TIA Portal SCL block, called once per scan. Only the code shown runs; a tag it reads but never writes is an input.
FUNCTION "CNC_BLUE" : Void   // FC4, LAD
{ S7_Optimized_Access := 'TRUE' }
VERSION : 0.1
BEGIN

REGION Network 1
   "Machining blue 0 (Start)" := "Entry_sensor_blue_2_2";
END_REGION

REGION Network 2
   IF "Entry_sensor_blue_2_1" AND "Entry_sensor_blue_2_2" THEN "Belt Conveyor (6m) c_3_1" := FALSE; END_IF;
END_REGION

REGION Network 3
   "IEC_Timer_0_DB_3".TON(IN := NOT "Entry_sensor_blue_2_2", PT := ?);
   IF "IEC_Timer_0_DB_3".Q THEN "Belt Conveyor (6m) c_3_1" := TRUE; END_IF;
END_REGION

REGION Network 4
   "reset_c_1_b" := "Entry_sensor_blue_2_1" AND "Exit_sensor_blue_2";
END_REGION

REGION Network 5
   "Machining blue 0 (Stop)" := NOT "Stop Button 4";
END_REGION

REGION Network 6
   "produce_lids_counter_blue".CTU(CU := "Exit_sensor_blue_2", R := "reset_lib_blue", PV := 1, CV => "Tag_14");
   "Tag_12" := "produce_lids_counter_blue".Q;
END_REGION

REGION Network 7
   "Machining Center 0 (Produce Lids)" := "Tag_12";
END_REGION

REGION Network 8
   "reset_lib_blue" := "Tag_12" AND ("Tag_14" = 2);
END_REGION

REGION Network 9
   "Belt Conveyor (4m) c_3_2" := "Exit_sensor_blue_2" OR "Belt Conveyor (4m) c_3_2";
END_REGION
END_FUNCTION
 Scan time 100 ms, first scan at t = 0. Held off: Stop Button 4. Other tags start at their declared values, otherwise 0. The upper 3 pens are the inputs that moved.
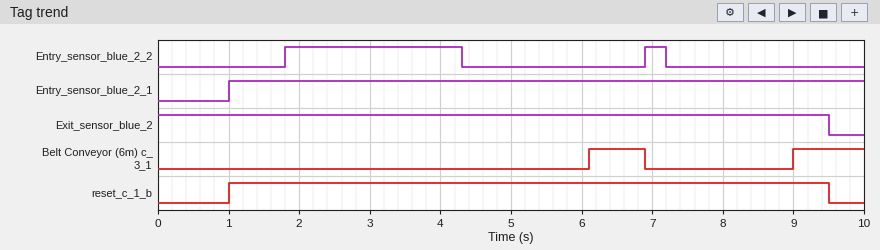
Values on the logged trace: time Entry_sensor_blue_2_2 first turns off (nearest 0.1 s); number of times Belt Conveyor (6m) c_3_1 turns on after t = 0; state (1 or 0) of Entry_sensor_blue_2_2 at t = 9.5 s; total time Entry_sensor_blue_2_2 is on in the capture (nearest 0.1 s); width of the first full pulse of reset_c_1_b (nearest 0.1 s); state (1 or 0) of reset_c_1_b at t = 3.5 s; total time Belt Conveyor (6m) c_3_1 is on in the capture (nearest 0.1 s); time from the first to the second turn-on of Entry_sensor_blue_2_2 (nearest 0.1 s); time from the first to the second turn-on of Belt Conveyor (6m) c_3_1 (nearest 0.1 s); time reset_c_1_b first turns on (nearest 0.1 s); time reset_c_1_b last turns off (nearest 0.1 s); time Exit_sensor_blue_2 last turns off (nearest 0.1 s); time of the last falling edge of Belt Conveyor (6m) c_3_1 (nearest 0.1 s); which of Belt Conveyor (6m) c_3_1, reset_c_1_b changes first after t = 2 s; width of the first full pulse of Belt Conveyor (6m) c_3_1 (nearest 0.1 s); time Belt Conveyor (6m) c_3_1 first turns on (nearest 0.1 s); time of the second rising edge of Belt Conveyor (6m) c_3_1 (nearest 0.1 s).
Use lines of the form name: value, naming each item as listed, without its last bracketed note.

time Entry_sensor_blue_2_2 first turns off: 4.3 s
number of times Belt Conveyor (6m) c_3_1 turns on after t = 0: 2
state (1 or 0) of Entry_sensor_blue_2_2 at t = 9.5 s: 0
total time Entry_sensor_blue_2_2 is on in the capture: 2.8 s
width of the first full pulse of reset_c_1_b: 8.5 s
state (1 or 0) of reset_c_1_b at t = 3.5 s: 1
total time Belt Conveyor (6m) c_3_1 is on in the capture: 1.8 s
time from the first to the second turn-on of Entry_sensor_blue_2_2: 5.1 s
time from the first to the second turn-on of Belt Conveyor (6m) c_3_1: 2.9 s
time reset_c_1_b first turns on: 1.0 s
time reset_c_1_b last turns off: 9.5 s
time Exit_sensor_blue_2 last turns off: 9.5 s
time of the last falling edge of Belt Conveyor (6m) c_3_1: 6.9 s
which of Belt Conveyor (6m) c_3_1, reset_c_1_b changes first after t = 2 s: Belt Conveyor (6m) c_3_1
width of the first full pulse of Belt Conveyor (6m) c_3_1: 0.8 s
time Belt Conveyor (6m) c_3_1 first turns on: 6.1 s
time of the second rising edge of Belt Conveyor (6m) c_3_1: 9.0 s
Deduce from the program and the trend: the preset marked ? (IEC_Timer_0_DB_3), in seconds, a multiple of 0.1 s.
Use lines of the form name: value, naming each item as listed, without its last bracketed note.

the preset marked ? (IEC_Timer_0_DB_3), in seconds, a multiple of 0.1 s: 1.8 s
